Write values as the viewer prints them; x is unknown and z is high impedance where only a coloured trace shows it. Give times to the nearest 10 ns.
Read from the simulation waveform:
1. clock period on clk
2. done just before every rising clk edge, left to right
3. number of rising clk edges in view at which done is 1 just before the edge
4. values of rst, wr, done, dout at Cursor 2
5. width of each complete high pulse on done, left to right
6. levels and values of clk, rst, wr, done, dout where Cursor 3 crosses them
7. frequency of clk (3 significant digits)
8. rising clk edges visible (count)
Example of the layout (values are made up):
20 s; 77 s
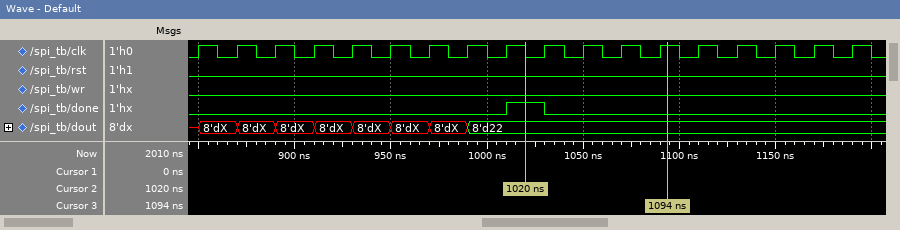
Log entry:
20 ns; 0 0 0 0 0 0 0 0 0 1 0 0 0 0 0 0 0 0; 1; rst=0, wr=0, done=1, dout=8'd22; 20 ns; clk=1, rst=0, wr=0, done=0, dout=8'd22; 50.0 MHz; 18
